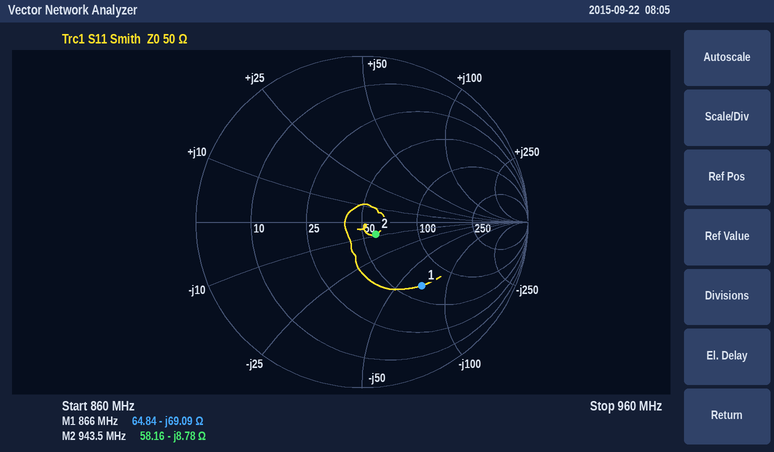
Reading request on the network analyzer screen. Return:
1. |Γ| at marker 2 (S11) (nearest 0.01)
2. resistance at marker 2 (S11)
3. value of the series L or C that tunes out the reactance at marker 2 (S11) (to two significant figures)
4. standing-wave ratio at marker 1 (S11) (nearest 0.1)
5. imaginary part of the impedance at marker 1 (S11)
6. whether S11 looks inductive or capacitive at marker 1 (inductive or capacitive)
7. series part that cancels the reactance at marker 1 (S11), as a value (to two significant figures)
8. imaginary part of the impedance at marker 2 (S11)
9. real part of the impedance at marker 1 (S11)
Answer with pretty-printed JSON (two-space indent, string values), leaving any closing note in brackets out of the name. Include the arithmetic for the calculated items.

{
  "|Γ| at marker 2 (S11)": "0.11",
  "resistance at marker 2": "58.16 Ω",
  "value of the series L or C that tunes out the reactance at marker 2 (S11)": "L = 8.78 Ω/(2π × 943.5 MHz) ≈ 1.5 nH",
  "standing-wave ratio at marker 1 (S11)": "3.2",
  "imaginary part of the impedance at marker 1": "-69.09 Ω",
  "whether S11 looks inductive or capacitive at marker 1": "capacitive",
  "series part that cancels the reactance at marker 1 (S11), as a value": "L = 69.09 Ω/(2π × 866 MHz) ≈ 13 nH",
  "imaginary part of the impedance at marker 2": "-8.78 Ω",
  "real part of the impedance at marker 1": "64.84 Ω"
}
